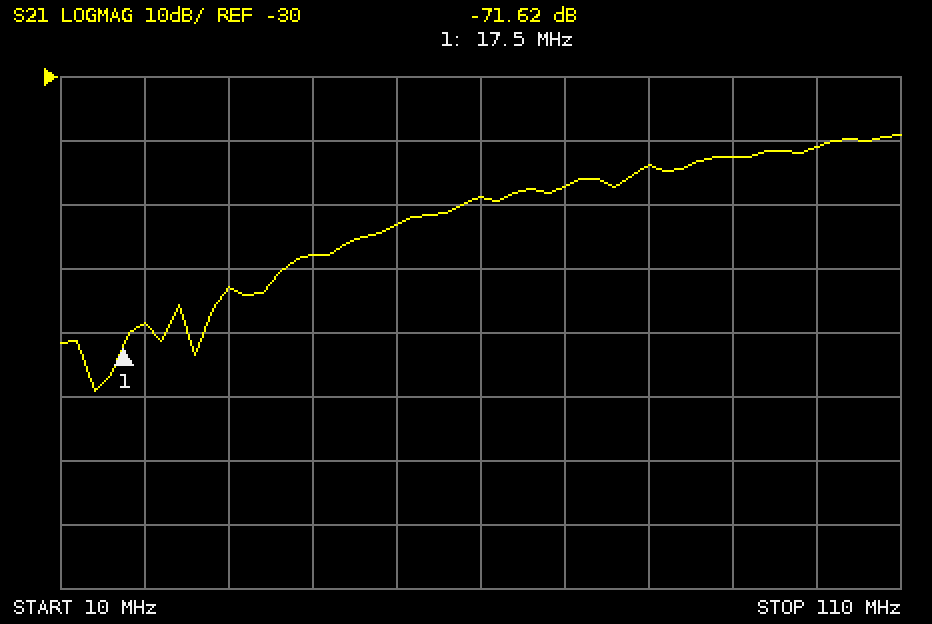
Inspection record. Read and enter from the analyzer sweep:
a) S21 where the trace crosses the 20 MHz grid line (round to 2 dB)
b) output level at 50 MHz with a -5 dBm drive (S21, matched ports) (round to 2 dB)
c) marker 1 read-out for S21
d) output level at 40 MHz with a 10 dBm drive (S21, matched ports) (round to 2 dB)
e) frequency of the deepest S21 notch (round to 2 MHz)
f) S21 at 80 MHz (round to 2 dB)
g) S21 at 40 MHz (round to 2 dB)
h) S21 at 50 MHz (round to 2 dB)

-68 dB
-58 dBm
-71.62 dB
-48 dBm
14 MHz
-44 dB
-58 dB
-54 dB
